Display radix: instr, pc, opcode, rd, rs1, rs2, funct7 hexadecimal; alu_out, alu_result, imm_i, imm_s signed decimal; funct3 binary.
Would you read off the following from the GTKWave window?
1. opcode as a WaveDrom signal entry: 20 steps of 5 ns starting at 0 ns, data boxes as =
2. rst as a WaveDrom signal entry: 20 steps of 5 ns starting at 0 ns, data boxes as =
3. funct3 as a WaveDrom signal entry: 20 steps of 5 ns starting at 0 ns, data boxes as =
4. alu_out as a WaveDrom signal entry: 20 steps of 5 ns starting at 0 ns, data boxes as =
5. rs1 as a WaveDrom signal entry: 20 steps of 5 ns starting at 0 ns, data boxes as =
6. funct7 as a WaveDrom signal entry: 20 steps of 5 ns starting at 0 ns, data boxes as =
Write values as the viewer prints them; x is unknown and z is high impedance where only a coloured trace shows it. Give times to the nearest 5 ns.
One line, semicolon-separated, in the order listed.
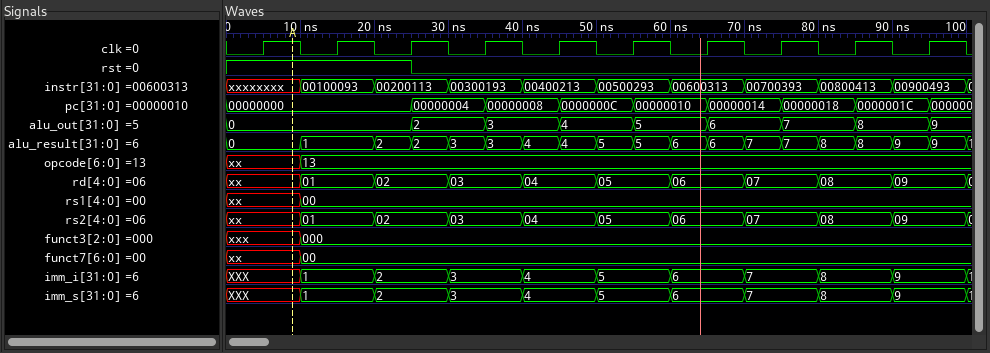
{name: 'opcode', wave: 'x.=.................', data: '13'}; {name: 'rst', wave: '1....0..............'}; {name: 'funct3', wave: 'x.=.................', data: '000'}; {name: 'alu_out', wave: '=....=.=.=.=.=.=.=.=', data: '0 2 3 4 5 6 7 8 9'}; {name: 'rs1', wave: 'x.=.................', data: '00'}; {name: 'funct7', wave: 'x.=.................', data: '00'}
